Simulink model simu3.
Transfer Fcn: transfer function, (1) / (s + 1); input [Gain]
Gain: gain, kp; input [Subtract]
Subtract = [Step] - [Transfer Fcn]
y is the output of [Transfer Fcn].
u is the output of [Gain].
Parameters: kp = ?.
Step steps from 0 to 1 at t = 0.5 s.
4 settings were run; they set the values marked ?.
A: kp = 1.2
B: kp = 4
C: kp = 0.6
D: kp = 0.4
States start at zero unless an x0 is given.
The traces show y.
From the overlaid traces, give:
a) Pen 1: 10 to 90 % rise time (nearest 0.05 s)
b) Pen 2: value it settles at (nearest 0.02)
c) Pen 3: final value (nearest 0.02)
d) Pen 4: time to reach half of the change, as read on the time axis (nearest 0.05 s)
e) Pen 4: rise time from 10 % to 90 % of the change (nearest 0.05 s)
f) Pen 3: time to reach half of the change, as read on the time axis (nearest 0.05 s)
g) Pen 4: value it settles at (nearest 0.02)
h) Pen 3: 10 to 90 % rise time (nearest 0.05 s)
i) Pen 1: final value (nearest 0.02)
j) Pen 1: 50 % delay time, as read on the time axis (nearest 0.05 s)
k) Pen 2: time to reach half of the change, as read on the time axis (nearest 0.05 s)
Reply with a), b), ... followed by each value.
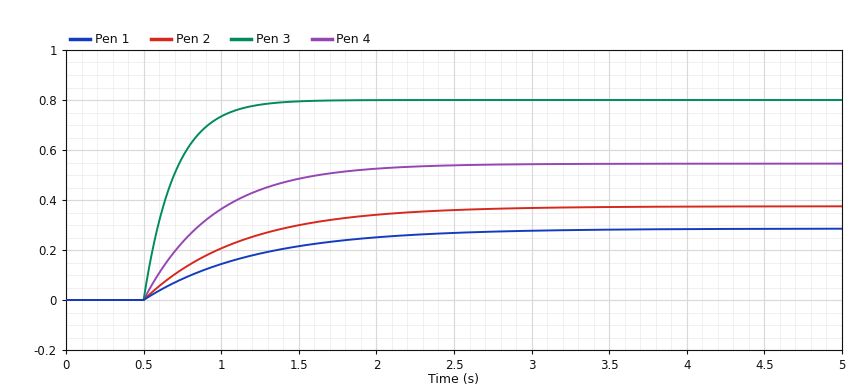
a) 1.55 s
b) 0.38
c) 0.80
d) 0.80 s
e) 1.00 s
f) 0.65 s
g) 0.54
h) 0.45 s
i) 0.28
j) 1.00 s
k) 0.95 s
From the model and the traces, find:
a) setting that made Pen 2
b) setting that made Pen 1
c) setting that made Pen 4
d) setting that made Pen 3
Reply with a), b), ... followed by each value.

a) C
b) D
c) A
d) B
